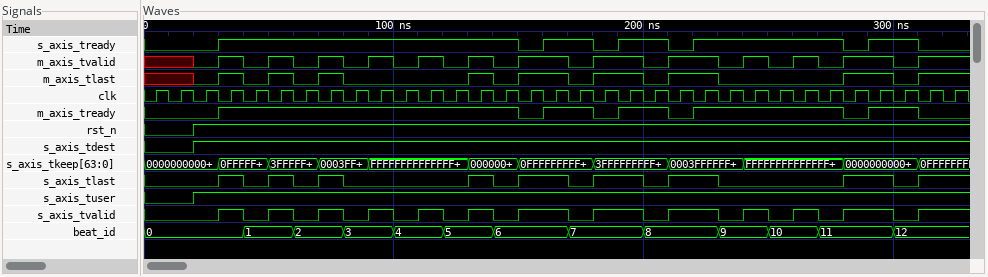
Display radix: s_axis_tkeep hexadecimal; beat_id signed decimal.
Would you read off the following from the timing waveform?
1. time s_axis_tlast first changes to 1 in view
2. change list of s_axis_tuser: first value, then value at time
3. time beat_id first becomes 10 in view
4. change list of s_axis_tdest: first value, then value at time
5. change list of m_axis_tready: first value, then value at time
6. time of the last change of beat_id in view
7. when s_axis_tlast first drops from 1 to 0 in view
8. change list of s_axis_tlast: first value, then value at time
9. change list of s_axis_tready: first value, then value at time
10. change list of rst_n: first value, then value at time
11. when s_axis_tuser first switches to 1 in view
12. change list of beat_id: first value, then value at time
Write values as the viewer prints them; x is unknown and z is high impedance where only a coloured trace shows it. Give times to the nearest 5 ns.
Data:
30 ns
0, 1 at 20 ns
250 ns
0, 1 at 20 ns
0, 1 at 30 ns, 0 at 150 ns, 1 at 160 ns, 0 at 180 ns, 1 at 190 ns, 0 at 210 ns, 1 at 220 ns, 0 at 280 ns, 1 at 290 ns, 0 at 310 ns
300 ns
40 ns
0, 1 at 30 ns, 0 at 40 ns, 1 at 50 ns, 0 at 60 ns, 1 at 70 ns, 0 at 80 ns, 1 at 130 ns, 0 at 140 ns, 1 at 150 ns, 0 at 170 ns, 1 at 180 ns, 0 at 200 ns, 1 at 210 ns, 0 at 230 ns, 1 at 280 ns, 0 at 300 ns, 1 at 310 ns
0, 1 at 30 ns, 0 at 150 ns, 1 at 160 ns, 0 at 180 ns, 1 at 190 ns, 0 at 210 ns, 1 at 220 ns, 0 at 280 ns, 1 at 290 ns, 0 at 310 ns
0, 1 at 20 ns
20 ns
0, 1 at 40 ns, 2 at 60 ns, 3 at 80 ns, 4 at 100 ns, 5 at 120 ns, 6 at 140 ns, 7 at 170 ns, 8 at 200 ns, 9 at 230 ns, 10 at 250 ns, 11 at 270 ns, 12 at 300 ns
